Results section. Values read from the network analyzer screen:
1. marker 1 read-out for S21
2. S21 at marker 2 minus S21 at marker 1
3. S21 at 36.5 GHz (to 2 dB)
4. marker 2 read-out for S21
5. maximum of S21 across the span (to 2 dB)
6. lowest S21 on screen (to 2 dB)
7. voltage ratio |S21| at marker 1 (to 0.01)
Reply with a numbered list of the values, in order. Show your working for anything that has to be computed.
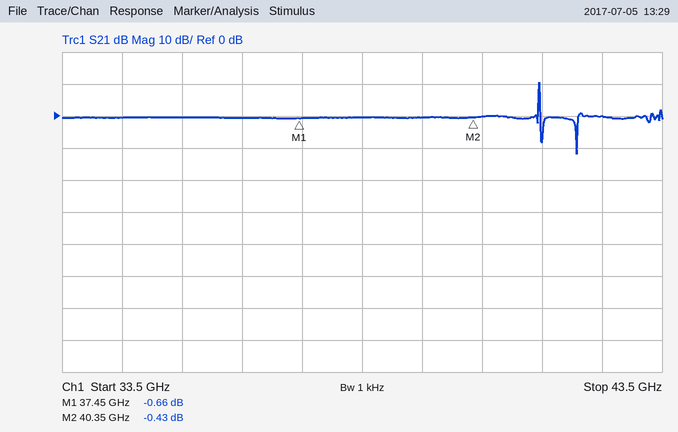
1. -0.66 dB
2. -0.43 − (-0.66) = 0.23 dB
3. 0 dB
4. -0.43 dB
5. 10 dB
6. -12 dB
7. 10^(-0.66/20) ≈ 0.93
